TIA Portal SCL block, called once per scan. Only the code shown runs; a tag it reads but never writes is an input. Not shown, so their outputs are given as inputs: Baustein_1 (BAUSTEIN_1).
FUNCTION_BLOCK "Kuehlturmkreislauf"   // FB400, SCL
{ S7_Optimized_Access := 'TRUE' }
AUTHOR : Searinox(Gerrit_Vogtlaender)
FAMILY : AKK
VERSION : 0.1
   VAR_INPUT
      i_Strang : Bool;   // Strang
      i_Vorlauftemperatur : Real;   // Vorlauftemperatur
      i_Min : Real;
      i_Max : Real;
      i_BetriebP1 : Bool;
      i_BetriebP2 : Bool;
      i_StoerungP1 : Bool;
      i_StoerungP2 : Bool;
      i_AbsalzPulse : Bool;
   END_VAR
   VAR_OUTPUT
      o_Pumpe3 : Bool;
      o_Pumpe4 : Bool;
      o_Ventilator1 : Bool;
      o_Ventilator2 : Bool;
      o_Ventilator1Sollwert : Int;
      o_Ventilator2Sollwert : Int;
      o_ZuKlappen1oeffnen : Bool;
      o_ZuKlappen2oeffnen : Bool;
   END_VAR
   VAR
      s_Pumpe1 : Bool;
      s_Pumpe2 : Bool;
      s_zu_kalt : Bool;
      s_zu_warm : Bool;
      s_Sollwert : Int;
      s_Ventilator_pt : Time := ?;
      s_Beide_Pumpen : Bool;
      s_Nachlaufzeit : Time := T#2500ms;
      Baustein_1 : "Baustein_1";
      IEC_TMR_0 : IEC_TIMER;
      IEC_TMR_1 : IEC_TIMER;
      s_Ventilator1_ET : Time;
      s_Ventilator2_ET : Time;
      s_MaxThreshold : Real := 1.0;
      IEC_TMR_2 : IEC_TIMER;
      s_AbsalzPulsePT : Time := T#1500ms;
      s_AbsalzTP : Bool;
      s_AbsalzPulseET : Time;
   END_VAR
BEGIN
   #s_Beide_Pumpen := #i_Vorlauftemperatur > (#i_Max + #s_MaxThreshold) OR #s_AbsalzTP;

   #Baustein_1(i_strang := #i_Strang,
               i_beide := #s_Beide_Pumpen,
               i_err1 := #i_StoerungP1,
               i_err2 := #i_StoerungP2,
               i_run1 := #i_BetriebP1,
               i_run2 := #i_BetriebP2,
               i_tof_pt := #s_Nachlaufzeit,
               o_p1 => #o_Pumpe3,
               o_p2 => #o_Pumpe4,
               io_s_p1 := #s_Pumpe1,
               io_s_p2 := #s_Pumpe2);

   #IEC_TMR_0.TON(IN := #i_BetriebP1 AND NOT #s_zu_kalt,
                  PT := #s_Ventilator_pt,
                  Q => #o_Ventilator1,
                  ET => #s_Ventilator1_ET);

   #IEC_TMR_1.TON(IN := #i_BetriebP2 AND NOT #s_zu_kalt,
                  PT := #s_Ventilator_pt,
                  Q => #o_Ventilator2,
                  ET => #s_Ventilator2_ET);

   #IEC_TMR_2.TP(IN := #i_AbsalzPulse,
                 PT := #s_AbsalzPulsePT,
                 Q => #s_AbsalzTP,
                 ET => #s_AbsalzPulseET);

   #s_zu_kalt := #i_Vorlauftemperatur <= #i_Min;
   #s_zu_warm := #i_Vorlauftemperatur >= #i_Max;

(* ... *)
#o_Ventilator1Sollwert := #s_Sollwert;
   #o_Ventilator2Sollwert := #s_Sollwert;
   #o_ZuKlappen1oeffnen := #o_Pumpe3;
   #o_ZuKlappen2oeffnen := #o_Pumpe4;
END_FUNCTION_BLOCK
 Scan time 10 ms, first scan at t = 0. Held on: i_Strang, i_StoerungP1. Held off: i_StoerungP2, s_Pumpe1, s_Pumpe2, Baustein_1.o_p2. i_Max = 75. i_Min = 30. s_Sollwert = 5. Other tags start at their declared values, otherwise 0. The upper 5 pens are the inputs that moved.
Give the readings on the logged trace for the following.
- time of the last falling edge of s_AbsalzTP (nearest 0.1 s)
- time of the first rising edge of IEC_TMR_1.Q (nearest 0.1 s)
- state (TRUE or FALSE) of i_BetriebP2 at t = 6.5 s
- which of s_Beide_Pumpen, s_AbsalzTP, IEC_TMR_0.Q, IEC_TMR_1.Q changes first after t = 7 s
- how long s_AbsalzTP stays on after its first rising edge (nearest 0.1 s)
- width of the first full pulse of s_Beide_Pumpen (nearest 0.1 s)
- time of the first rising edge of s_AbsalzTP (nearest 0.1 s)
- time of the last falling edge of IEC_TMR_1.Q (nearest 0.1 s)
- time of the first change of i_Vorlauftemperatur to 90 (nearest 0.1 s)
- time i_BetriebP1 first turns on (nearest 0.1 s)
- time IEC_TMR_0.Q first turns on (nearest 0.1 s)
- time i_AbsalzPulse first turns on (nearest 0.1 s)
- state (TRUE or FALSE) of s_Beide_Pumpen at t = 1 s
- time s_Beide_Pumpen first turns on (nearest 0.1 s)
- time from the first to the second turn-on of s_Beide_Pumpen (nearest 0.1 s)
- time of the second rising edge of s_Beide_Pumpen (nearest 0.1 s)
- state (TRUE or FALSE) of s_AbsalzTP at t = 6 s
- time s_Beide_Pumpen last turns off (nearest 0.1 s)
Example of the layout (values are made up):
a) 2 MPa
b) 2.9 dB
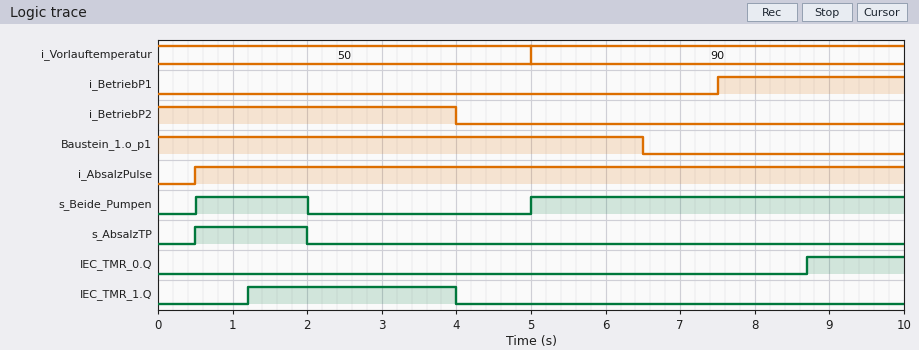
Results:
a) 2.0 s
b) 1.2 s
c) FALSE
d) IEC_TMR_0.Q
e) 1.5 s
f) 1.5 s
g) 0.5 s
h) 4.0 s
i) 5.0 s
j) 7.5 s
k) 8.7 s
l) 0.5 s
m) TRUE
n) 0.5 s
o) 4.5 s
p) 5.0 s
q) FALSE
r) 2.0 s
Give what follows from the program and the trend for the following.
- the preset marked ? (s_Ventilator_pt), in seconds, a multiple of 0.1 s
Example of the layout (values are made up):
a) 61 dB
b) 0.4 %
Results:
a) 1.2 s
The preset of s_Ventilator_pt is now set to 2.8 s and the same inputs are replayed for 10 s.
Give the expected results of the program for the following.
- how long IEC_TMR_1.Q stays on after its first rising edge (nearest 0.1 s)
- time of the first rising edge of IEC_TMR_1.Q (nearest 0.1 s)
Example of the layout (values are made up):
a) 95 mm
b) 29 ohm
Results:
a) 1.2 s
b) 2.8 s
